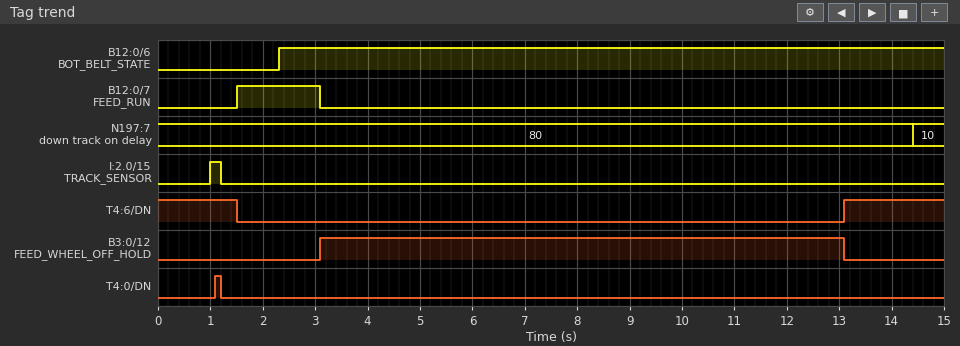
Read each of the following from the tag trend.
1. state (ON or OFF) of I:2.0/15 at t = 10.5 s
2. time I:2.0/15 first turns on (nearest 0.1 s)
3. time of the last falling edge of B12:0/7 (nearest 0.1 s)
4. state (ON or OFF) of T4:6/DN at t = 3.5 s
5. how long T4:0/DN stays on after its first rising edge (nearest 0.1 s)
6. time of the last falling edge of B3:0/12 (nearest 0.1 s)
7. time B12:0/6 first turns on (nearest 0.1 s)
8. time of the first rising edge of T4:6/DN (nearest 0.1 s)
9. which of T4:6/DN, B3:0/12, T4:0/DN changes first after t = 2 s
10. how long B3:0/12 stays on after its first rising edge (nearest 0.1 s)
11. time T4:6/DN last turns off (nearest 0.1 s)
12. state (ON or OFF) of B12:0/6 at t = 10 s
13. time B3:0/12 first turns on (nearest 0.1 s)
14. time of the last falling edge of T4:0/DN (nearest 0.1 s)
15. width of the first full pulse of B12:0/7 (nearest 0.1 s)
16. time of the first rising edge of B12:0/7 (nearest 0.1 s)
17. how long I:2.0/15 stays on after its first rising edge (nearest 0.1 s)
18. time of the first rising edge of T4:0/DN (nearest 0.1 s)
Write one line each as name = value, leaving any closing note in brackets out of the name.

state (ON or OFF) of I:2.0/15 at t = 10.5 s = OFF
time I:2.0/15 first turns on = 1.0 s
time of the last falling edge of B12:0/7 = 3.1 s
state (ON or OFF) of T4:6/DN at t = 3.5 s = OFF
how long T4:0/DN stays on after its first rising edge = 0.1 s
time of the last falling edge of B3:0/12 = 13.1 s
time B12:0/6 first turns on = 2.3 s
time of the first rising edge of T4:6/DN = 13.1 s
which of T4:6/DN, B3:0/12, T4:0/DN changes first after t = 2 s = B3:0/12
how long B3:0/12 stays on after its first rising edge = 10.0 s
time T4:6/DN last turns off = 1.5 s
state (ON or OFF) of B12:0/6 at t = 10 s = ON
time B3:0/12 first turns on = 3.1 s
time of the last falling edge of T4:0/DN = 1.2 s
width of the first full pulse of B12:0/7 = 1.6 s
time of the first rising edge of B12:0/7 = 1.5 s
how long I:2.0/15 stays on after its first rising edge = 0.2 s
time of the first rising edge of T4:0/DN = 1.1 s
